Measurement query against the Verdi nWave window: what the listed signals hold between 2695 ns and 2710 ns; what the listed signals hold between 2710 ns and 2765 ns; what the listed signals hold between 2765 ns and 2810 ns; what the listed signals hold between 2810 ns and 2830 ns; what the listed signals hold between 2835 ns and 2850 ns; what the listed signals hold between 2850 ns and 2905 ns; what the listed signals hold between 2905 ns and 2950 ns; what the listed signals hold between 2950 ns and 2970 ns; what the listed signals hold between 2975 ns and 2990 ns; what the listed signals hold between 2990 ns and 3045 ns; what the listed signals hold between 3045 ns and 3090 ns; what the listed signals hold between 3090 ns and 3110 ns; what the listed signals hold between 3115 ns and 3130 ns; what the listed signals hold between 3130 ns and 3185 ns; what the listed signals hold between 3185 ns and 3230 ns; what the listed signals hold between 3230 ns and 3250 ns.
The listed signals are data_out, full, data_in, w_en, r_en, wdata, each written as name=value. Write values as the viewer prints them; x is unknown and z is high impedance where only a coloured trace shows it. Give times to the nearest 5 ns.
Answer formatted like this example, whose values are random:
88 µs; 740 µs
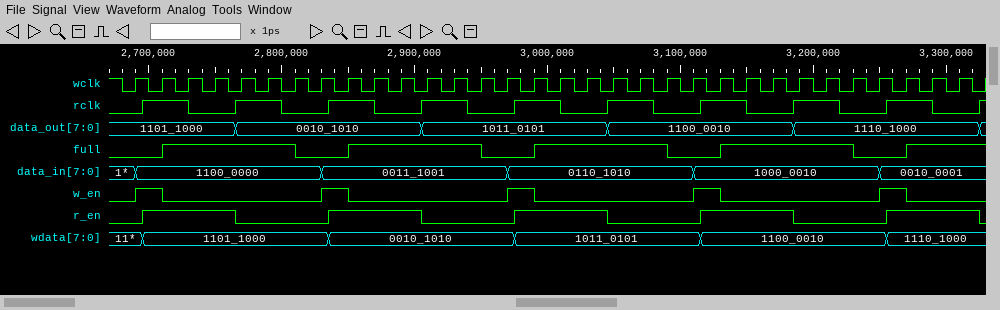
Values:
data_out=1101_1000, full=0, data_in=1100_0000, w_en=1, r_en=1, wdata=1101_1000; data_out=1101_1000, full=1, data_in=1100_0000, w_en=0, r_en=1, wdata=1101_1000; data_out=0010_1010, full=1, data_in=1100_0000, w_en=0, r_en=0, wdata=1101_1000; data_out=0010_1010, full=0, data_in=1100_0000, w_en=0, r_en=0, wdata=1101_1000; data_out=0010_1010, full=0, data_in=0011_1001, w_en=1, r_en=1, wdata=0010_1010; data_out=0010_1010, full=1, data_in=0011_1001, w_en=0, r_en=1, wdata=0010_1010; data_out=1011_0101, full=1, data_in=0011_1001, w_en=0, r_en=0, wdata=0010_1010; data_out=1011_0101, full=0, data_in=0011_1001, w_en=0, r_en=0, wdata=0010_1010; data_out=1011_0101, full=0, data_in=0110_1010, w_en=1, r_en=1, wdata=1011_0101; data_out=1011_0101, full=1, data_in=0110_1010, w_en=0, r_en=1, wdata=1011_0101; data_out=1100_0010, full=1, data_in=0110_1010, w_en=0, r_en=0, wdata=1011_0101; data_out=1100_0010, full=0, data_in=0110_1010, w_en=0, r_en=0, wdata=1011_0101; data_out=1100_0010, full=0, data_in=1000_0010, w_en=1, r_en=1, wdata=1100_0010; data_out=1100_0010, full=1, data_in=1000_0010, w_en=0, r_en=1, wdata=1100_0010; data_out=1110_1000, full=1, data_in=1000_0010, w_en=0, r_en=0, wdata=1100_0010; data_out=1110_1000, full=0, data_in=1000_0010, w_en=0, r_en=0, wdata=1100_0010
